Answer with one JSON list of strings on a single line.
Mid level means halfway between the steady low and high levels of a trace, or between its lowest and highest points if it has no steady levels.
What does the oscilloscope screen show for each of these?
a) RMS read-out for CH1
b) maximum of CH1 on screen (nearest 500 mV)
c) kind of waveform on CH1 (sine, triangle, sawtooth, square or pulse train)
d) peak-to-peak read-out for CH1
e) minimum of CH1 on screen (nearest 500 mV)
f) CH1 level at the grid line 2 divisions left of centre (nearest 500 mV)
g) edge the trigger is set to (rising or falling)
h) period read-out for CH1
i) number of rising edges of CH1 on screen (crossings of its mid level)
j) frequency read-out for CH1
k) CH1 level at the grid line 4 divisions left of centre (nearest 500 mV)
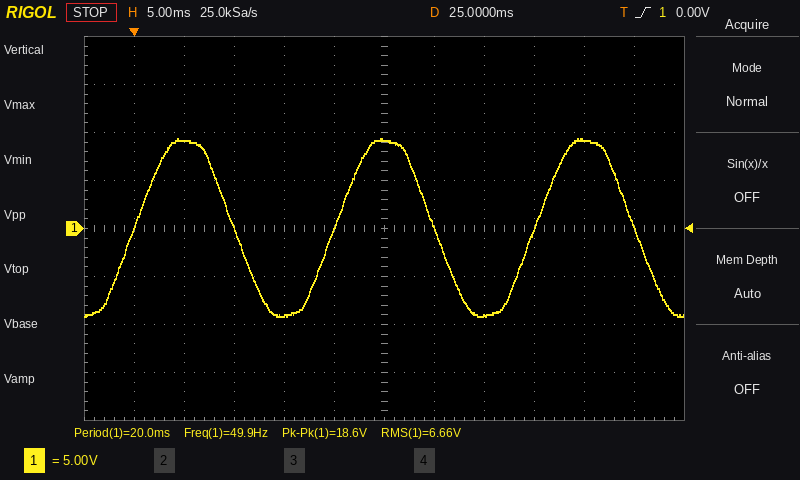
["6.66 V", "9.5 V", "sine", "18.6 V", "-9.0 V", "-9.0 V", "rising", "20.0 ms", "3", "49.9 Hz", "9.0 V"]
